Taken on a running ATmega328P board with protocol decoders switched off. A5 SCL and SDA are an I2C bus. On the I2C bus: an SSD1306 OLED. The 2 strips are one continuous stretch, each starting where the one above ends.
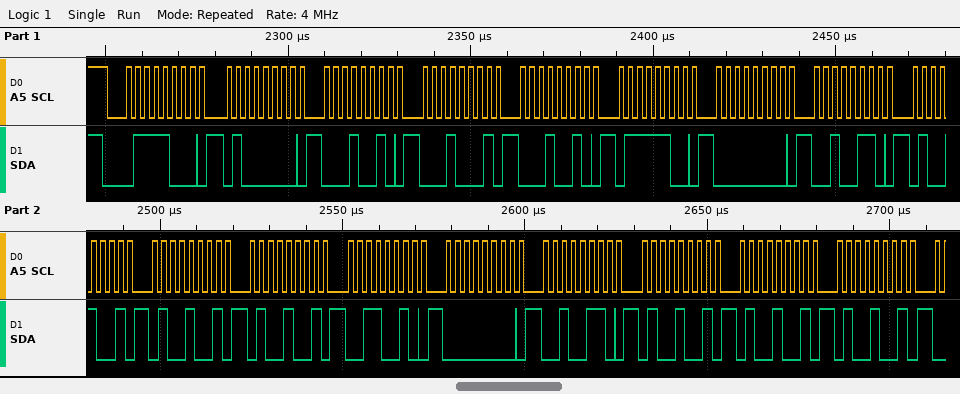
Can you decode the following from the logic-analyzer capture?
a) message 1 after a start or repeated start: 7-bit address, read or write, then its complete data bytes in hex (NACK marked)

0x3C write: 40 12 11 12 7C 00 26 49 49 49 32 00 26 49 49 49
